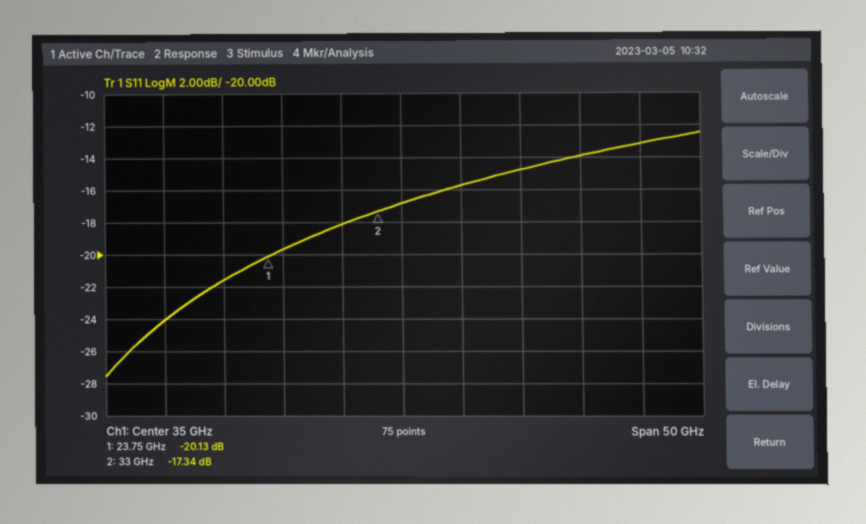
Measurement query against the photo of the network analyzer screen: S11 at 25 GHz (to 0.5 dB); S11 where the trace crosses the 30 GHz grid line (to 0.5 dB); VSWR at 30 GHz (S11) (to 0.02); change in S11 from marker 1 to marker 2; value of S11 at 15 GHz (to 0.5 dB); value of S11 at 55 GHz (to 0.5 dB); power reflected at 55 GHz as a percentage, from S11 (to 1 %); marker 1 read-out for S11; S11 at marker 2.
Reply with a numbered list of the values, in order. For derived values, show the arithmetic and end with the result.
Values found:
1. -19.5 dB
2. -18.0 dB
3. |Γ| = 10^(-18/20) = 0.1259; VSWR = (1 + 0.1259)/(1 − 0.1259) ≈ 1.29, so 1.28 to the nearest 0.02
4. -17.34 − (-20.13) = 2.79 dB
5. -24.0 dB
6. -13.0 dB
7. 10^(-13/10) ≈ 5 %
8. -20.13 dB
9. -17.34 dB
